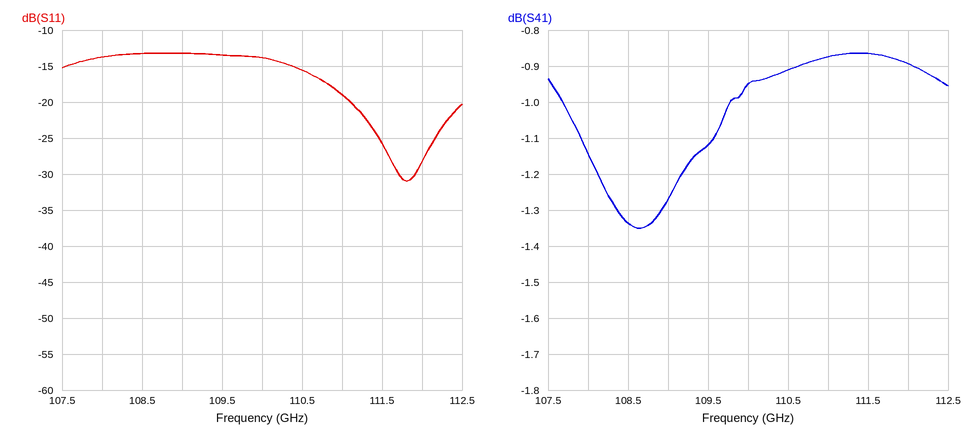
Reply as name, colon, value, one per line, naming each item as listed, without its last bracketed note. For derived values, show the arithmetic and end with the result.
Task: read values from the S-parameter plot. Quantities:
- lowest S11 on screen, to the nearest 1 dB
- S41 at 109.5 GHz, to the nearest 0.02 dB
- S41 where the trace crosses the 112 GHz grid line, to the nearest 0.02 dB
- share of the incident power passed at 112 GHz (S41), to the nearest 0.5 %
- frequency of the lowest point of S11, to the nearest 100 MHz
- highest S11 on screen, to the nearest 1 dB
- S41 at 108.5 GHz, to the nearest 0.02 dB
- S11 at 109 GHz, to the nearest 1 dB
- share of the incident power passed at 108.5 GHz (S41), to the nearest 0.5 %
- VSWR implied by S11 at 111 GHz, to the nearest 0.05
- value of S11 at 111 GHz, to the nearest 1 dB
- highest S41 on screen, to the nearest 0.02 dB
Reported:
lowest S11 on screen, to the nearest 1 dB: -31 dB
S41 at 109.5 GHz, to the nearest 0.02 dB: -1.12 dB
S41 where the trace crosses the 112 GHz grid line, to the nearest 0.02 dB: -0.90 dB
share of the incident power passed at 112 GHz (S41), to the nearest 0.5 %: 10^(-0.9/10) ≈ 81.3 %, so 81.5 % to the nearest 0.5 %
frequency of the lowest point of S11, to the nearest 100 MHz: 111.8 GHz
highest S11 on screen, to the nearest 1 dB: -13 dB
S41 at 108.5 GHz, to the nearest 0.02 dB: -1.34 dB
S11 at 109 GHz, to the nearest 1 dB: -13 dB
share of the incident power passed at 108.5 GHz (S41), to the nearest 0.5 %: 10^(-1.34/10) ≈ 73.5 %
VSWR implied by S11 at 111 GHz, to the nearest 0.05: |Γ| = 10^(-19/20) = 0.1122; VSWR = (1 + 0.1122)/(1 − 0.1122) ≈ 1.25
value of S11 at 111 GHz, to the nearest 1 dB: -19 dB
highest S41 on screen, to the nearest 0.02 dB: -0.86 dB
